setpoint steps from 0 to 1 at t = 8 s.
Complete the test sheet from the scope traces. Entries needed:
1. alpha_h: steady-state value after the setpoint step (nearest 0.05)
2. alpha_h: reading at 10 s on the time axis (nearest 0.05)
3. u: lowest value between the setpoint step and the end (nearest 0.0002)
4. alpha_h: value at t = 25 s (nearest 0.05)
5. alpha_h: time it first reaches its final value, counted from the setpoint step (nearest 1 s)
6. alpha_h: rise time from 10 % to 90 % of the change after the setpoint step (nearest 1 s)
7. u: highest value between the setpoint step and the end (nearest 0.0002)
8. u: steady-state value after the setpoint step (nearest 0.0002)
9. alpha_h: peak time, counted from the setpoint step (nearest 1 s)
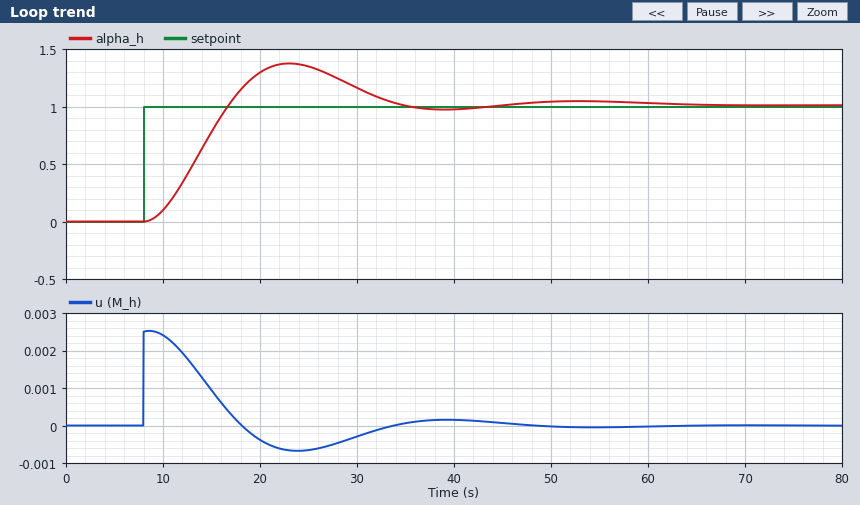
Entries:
1.00
0.10
-0.0006
1.35
9 s
6 s
0.0026
0.0000
15 s
